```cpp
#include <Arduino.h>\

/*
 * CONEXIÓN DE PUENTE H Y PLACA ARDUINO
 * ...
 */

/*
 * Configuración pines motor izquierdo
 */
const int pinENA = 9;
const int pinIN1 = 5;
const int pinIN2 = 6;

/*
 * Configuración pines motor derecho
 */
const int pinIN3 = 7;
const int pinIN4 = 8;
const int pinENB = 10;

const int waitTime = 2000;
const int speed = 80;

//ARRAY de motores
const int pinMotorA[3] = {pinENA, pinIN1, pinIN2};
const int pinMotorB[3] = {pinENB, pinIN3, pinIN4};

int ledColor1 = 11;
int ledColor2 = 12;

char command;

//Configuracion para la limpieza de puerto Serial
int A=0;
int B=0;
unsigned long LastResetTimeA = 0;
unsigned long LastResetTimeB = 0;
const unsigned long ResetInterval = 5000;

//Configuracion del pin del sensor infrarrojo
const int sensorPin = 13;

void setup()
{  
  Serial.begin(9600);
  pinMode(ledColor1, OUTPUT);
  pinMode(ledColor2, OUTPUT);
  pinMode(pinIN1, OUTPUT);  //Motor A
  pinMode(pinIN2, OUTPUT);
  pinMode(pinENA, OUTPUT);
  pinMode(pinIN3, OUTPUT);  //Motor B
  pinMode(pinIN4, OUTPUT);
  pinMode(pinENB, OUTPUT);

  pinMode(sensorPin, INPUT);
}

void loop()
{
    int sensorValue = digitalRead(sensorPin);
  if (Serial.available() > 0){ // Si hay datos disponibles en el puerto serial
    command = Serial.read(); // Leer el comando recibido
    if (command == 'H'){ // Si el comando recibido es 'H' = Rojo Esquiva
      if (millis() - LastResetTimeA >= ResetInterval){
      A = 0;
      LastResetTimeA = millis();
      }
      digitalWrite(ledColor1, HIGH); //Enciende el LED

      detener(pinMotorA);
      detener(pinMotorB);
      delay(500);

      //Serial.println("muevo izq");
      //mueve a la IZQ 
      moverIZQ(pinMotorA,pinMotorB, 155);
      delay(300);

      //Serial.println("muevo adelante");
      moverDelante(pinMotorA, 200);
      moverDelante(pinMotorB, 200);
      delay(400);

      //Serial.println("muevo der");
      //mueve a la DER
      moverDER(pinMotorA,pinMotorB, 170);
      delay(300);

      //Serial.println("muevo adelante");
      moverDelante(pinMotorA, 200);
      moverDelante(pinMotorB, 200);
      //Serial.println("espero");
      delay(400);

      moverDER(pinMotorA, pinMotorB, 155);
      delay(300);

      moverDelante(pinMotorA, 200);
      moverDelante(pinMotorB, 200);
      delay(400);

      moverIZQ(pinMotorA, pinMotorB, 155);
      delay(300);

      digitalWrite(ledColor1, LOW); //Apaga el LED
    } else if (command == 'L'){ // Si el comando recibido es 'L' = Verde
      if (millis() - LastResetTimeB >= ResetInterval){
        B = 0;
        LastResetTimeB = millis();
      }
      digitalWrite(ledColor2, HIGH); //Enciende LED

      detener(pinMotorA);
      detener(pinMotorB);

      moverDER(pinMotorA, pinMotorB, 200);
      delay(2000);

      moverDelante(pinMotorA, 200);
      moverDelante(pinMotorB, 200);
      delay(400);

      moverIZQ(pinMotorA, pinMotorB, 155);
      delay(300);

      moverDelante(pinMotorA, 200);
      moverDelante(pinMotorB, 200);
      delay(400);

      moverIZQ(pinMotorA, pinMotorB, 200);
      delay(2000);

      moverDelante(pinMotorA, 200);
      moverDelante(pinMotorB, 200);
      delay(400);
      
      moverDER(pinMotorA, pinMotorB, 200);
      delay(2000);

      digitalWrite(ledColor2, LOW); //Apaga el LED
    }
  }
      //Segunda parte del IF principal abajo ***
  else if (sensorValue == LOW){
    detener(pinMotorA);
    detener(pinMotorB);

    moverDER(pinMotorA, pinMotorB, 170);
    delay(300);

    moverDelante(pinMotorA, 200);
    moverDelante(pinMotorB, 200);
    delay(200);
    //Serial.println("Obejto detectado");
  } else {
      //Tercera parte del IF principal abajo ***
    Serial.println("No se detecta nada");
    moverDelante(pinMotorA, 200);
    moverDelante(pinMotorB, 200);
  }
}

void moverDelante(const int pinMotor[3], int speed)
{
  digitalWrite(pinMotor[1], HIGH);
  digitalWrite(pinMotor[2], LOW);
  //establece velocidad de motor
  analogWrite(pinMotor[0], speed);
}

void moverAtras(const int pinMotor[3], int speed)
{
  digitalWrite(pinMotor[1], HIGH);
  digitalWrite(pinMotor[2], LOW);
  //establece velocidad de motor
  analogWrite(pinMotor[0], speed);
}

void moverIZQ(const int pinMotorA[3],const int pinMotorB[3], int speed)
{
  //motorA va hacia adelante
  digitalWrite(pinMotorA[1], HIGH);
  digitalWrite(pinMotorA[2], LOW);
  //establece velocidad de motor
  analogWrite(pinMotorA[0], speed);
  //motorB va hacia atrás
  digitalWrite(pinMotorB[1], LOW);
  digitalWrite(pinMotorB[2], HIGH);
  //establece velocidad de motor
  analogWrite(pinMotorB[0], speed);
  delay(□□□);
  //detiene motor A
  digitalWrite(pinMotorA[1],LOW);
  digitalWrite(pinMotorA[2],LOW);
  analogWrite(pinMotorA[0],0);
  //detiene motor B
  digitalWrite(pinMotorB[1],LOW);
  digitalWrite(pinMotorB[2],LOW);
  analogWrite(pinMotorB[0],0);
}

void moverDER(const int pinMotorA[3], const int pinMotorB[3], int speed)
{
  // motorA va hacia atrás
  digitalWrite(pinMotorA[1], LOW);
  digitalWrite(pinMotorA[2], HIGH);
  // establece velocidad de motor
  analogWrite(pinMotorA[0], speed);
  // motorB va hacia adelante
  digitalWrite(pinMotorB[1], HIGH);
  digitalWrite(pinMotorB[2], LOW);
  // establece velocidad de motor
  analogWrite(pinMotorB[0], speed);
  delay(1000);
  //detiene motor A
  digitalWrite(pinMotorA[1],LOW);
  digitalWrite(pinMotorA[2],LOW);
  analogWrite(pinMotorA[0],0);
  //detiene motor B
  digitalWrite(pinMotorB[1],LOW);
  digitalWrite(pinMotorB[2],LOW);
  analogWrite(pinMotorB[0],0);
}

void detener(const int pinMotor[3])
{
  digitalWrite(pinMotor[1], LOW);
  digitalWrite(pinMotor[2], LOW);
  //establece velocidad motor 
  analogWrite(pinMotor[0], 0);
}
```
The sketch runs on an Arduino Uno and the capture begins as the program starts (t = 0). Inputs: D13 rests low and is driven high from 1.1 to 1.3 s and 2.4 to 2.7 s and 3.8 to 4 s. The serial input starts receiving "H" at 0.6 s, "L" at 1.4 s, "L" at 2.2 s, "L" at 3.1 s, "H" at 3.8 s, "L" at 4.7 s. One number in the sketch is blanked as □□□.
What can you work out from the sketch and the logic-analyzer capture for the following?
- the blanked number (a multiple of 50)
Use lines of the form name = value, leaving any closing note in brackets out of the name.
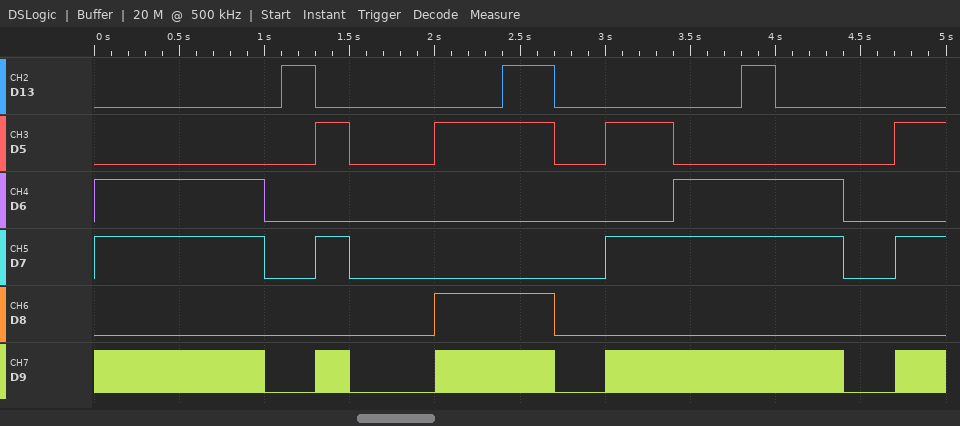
the blanked number = 700
